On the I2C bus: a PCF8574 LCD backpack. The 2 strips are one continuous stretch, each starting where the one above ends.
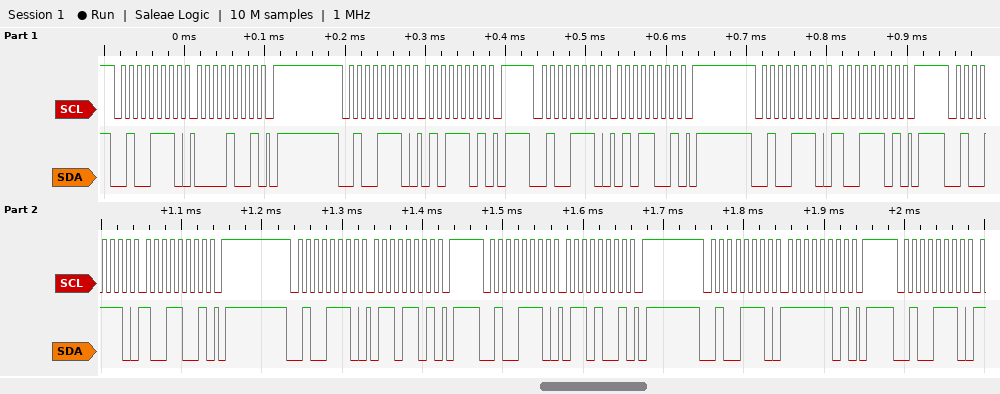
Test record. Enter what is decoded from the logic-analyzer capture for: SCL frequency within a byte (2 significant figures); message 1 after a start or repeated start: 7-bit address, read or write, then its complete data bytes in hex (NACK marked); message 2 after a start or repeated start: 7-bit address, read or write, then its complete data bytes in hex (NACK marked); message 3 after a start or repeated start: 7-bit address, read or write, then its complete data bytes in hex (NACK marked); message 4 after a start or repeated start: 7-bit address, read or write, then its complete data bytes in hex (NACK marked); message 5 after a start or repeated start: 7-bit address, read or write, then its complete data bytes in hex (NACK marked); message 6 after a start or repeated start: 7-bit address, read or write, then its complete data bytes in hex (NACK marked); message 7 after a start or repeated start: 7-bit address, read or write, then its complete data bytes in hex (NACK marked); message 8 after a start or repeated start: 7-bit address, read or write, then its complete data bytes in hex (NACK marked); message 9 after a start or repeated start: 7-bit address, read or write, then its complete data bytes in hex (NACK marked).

100 kHz
0x27 write: 09
0x27 write: 5D
0x27 write: 59
0x27 write: 9D
0x27 write: 99
0x27 write: 6D
0x27 write: 69
0x27 write: FD
0x27 write
